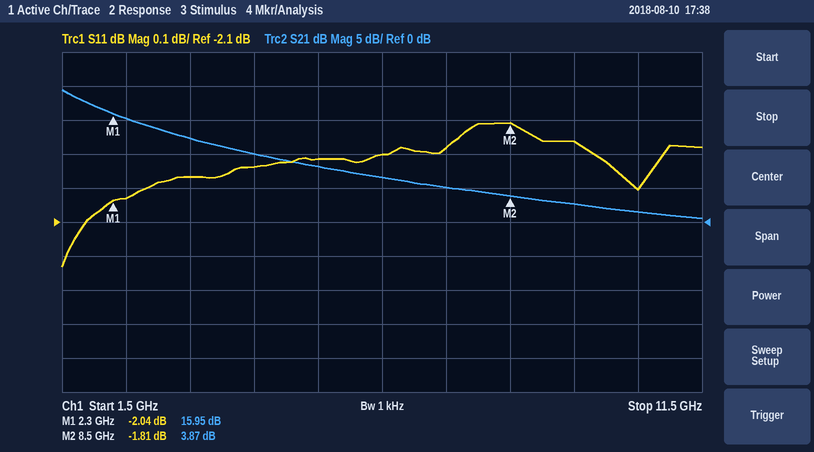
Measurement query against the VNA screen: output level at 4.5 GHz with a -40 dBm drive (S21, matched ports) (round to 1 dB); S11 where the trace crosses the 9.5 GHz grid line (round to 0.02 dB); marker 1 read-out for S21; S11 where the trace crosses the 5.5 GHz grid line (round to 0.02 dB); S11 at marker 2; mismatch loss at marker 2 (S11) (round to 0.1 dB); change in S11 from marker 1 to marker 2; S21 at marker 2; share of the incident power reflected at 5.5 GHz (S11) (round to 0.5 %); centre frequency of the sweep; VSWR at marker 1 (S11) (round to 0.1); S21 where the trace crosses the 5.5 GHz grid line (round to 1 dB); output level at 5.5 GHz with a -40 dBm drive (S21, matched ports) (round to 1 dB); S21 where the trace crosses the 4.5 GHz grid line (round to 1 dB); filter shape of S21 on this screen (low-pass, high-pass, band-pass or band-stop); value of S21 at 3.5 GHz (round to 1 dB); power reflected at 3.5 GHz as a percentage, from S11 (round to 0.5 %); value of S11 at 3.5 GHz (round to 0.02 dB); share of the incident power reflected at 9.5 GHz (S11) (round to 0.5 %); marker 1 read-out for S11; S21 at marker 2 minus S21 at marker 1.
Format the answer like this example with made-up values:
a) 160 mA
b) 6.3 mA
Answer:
a) -30 dBm
b) -1.86 dB
c) 15.95 dB
d) -1.92 dB
e) -1.81 dB
f) 4.7 dB
g) 0.23 dB
h) 3.87 dB
i) 64.5 %
j) 6.5 GHz
k) 8.6
l) 8 dB
m) -32 dBm
n) 10 dB
o) low-pass
p) 12 dB
q) 63.5 %
r) -1.96 dB
s) 65.0 %
t) -2.04 dB
u) -12.08 dB
